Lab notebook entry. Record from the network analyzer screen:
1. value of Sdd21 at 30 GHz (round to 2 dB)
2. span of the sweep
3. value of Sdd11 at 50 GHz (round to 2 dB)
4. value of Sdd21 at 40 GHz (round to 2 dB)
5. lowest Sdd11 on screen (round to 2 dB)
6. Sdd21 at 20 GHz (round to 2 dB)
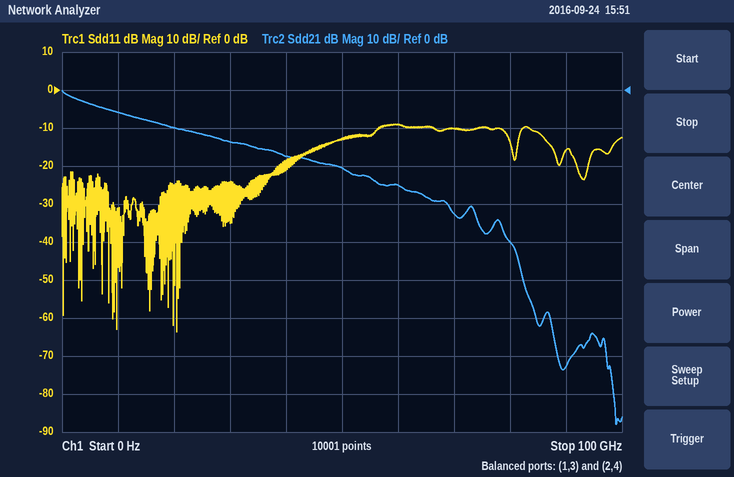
-14 dB
100 GHz
-12 dB
-18 dB
-64 dB
-10 dB
